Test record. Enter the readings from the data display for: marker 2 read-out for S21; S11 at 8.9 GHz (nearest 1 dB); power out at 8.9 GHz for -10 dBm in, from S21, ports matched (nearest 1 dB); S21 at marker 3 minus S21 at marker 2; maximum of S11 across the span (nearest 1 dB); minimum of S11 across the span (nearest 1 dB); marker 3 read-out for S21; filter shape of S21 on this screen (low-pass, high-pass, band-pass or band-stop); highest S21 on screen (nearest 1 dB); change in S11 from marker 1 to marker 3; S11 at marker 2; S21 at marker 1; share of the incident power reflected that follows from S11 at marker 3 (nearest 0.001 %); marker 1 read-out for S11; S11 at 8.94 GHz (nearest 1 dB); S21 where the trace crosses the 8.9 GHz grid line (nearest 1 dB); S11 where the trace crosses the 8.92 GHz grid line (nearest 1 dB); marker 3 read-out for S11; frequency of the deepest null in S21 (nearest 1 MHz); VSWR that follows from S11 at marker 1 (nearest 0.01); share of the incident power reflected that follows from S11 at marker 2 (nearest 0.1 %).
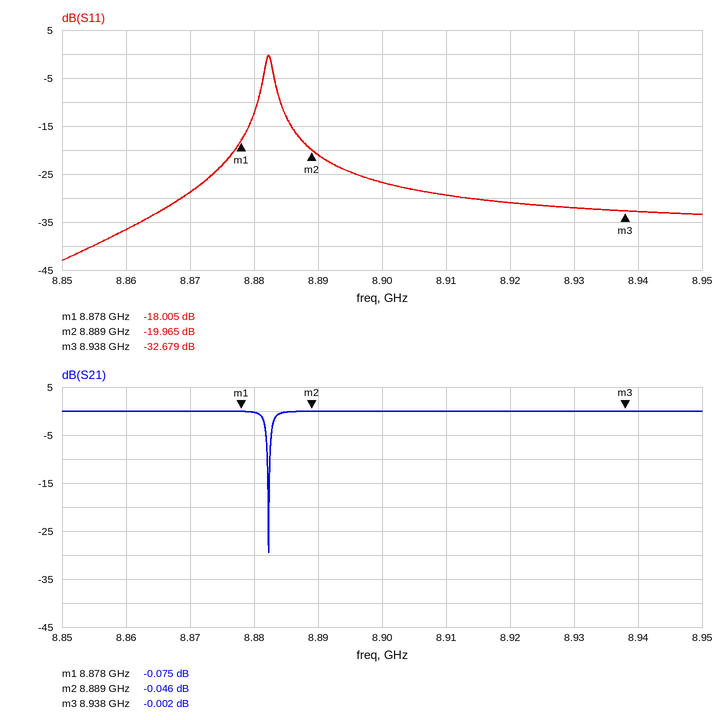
-0.046 dB
-27 dB
-10 dBm
0.044 dB
0 dB
-43 dB
-0.002 dB
band-stop
0 dB
-14.674 dB
-19.965 dB
-0.075 dB
0.054 %
-18.005 dB
-33 dB
0 dB
-31 dB
-32.679 dB
8.882 GHz
1.29
1.0 %
